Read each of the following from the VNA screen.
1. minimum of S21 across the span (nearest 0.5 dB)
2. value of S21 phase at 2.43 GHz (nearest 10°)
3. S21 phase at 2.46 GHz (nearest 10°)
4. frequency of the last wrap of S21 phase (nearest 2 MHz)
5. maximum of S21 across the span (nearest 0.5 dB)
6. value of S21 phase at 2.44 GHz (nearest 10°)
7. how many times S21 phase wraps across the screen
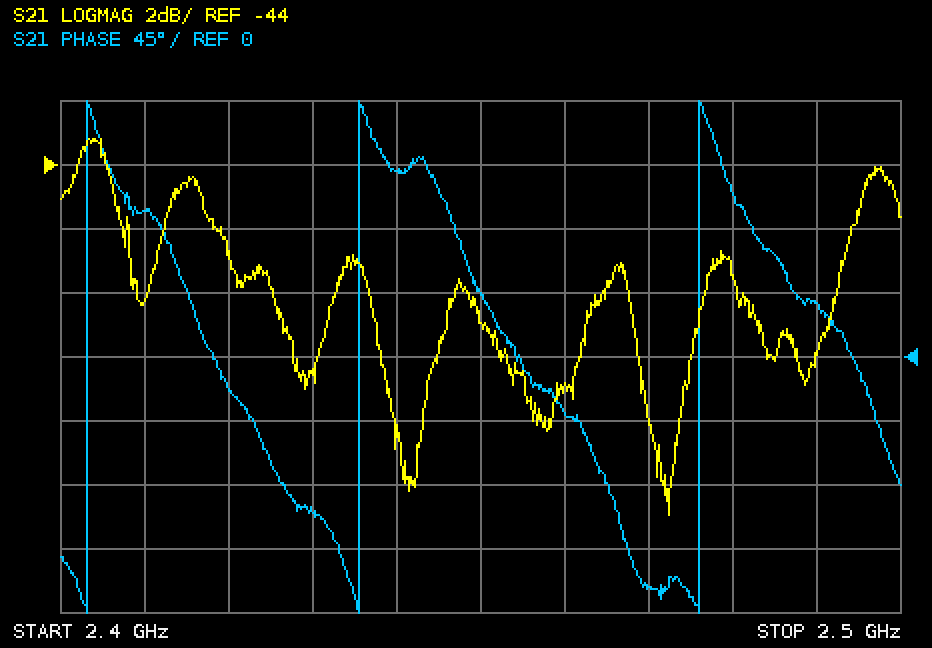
-55.0 dB
-110°
-40°
2.476 GHz
-43.0 dB
130°
3
